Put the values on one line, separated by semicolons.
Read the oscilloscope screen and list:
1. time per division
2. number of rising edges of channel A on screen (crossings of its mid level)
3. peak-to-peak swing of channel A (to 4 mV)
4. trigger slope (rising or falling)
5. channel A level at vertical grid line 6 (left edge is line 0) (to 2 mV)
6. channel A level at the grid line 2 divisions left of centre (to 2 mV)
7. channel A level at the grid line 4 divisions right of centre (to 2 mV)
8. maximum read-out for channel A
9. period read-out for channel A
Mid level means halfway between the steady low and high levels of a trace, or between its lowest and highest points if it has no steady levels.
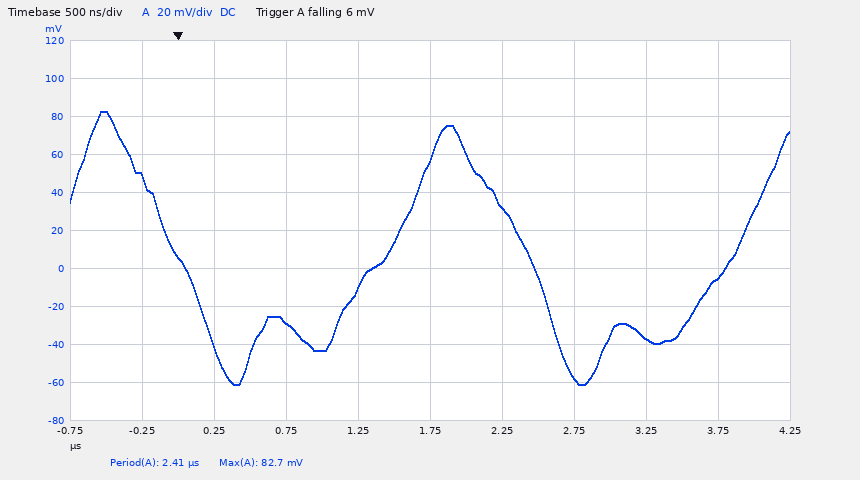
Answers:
500 ns; 2; 144 mV; falling; 32 mV; -28 mV; -4 mV; 82.7 mV; 2.41 µs
